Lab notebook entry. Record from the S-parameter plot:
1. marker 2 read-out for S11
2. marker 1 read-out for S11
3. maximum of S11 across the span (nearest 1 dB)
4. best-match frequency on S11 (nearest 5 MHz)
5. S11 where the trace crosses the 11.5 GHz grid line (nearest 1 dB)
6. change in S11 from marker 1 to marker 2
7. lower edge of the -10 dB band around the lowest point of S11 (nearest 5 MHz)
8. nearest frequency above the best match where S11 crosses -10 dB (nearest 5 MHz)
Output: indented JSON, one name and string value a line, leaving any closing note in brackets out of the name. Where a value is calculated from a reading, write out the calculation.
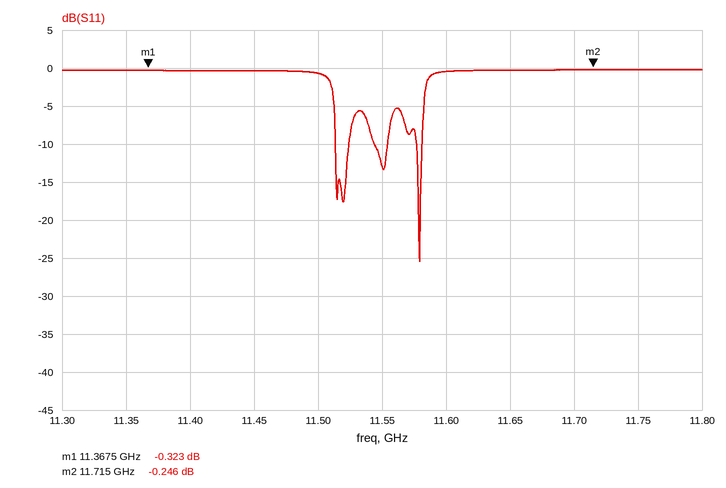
{
  "marker 2 read-out for S11": "-0.246 dB",
  "marker 1 read-out for S11": "-0.323 dB",
  "maximum of S11 across the span": "0 dB",
  "best-match frequency on S11": "11.580 GHz",
  "S11 where the trace crosses the 11.5 GHz grid line": "-1 dB",
  "change in S11 from marker 1 to marker 2": "-0.246 − (-0.323) = 0.077 dB",
  "lower edge of the -10 dB band around the lowest point of S11": "11.575 GHz",
  "nearest frequency above the best match where S11 crosses -10 dB": "11.580 GHz"
}
